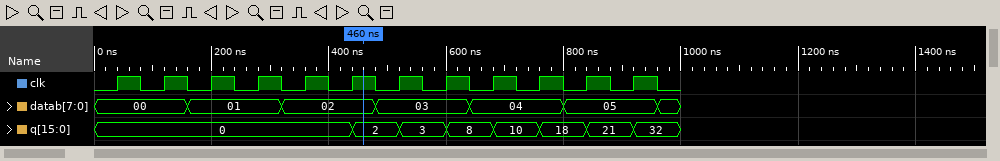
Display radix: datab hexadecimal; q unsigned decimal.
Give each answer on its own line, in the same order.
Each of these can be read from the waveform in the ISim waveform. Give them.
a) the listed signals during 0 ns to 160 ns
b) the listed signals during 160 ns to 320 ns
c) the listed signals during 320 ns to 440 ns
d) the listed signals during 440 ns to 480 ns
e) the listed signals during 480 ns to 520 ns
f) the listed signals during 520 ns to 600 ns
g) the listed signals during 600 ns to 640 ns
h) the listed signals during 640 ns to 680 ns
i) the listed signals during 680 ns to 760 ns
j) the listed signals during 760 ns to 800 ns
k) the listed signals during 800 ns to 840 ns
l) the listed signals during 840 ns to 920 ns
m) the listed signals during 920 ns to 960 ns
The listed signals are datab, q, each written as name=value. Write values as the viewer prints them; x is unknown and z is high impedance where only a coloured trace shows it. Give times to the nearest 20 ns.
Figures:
datab=00, q=0
datab=01, q=0
datab=02, q=0
datab=02, q=2
datab=03, q=2
datab=03, q=3
datab=03, q=8
datab=04, q=8
datab=04, q=10
datab=04, q=18
datab=05, q=18
datab=05, q=21
datab=05, q=32
